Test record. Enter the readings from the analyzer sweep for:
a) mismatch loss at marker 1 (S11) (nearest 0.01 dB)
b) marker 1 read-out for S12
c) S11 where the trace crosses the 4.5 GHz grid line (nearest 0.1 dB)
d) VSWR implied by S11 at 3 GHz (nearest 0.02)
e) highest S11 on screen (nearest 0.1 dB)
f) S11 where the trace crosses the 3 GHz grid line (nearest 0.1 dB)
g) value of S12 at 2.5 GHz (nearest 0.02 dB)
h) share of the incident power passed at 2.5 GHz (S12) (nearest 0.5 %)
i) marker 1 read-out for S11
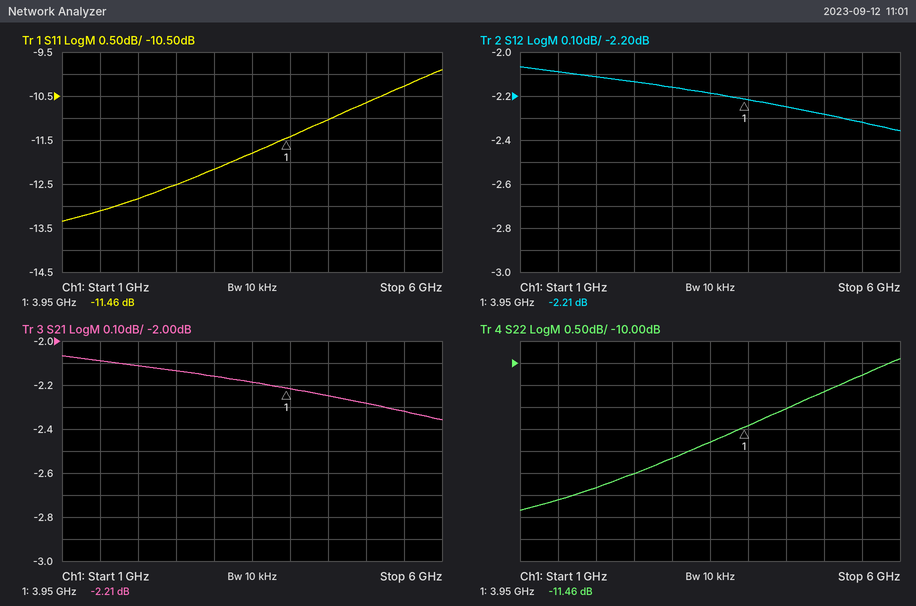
0.32 dB
-2.21 dB
-11.0 dB
1.66
-9.9 dB
-12.2 dB
-2.14 dB
61.0 %
-11.46 dB
